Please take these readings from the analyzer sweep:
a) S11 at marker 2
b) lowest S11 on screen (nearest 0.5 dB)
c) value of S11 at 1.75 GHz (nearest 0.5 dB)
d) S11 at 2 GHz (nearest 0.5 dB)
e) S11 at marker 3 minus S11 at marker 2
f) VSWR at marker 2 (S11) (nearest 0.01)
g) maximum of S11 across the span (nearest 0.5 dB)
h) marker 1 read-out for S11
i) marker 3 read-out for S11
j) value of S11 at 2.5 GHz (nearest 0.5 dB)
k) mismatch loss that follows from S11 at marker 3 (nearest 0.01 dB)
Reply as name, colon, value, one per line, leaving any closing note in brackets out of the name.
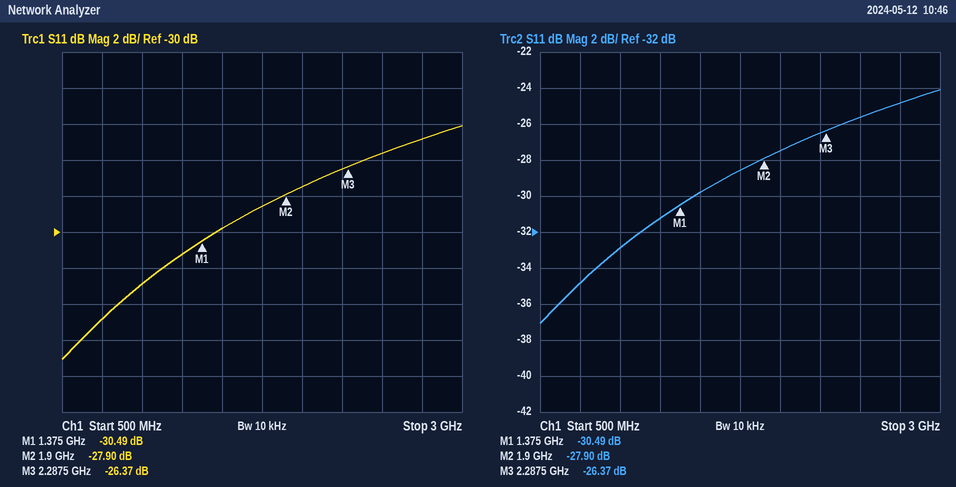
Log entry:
S11 at marker 2: -27.90 dB
lowest S11 on screen: -37.0 dB
value of S11 at 1.75 GHz: -28.5 dB
S11 at 2 GHz: -27.5 dB
S11 at marker 3 minus S11 at marker 2: 1.53 dB
VSWR at marker 2 (S11): 1.08
maximum of S11 across the span: -24.0 dB
marker 1 read-out for S11: -30.49 dB
marker 3 read-out for S11: -26.37 dB
value of S11 at 2.5 GHz: -25.5 dB
mismatch loss that follows from S11 at marker 3: 0.01 dB
